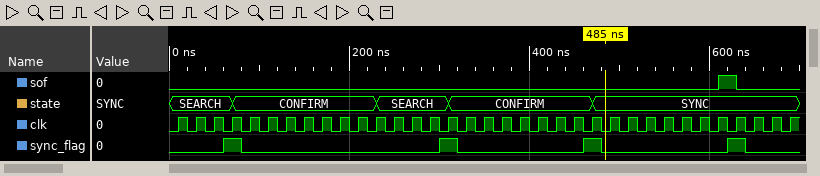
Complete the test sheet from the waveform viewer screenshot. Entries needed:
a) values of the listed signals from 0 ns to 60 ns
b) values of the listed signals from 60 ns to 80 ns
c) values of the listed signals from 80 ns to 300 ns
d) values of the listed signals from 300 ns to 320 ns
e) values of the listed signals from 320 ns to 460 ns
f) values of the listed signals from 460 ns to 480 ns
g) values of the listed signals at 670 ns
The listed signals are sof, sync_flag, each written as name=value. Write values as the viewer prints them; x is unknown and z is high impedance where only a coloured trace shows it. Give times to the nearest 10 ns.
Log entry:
sof=0, sync_flag=0
sof=0, sync_flag=1
sof=0, sync_flag=0
sof=0, sync_flag=1
sof=0, sync_flag=0
sof=0, sync_flag=1
sof=0, sync_flag=0
